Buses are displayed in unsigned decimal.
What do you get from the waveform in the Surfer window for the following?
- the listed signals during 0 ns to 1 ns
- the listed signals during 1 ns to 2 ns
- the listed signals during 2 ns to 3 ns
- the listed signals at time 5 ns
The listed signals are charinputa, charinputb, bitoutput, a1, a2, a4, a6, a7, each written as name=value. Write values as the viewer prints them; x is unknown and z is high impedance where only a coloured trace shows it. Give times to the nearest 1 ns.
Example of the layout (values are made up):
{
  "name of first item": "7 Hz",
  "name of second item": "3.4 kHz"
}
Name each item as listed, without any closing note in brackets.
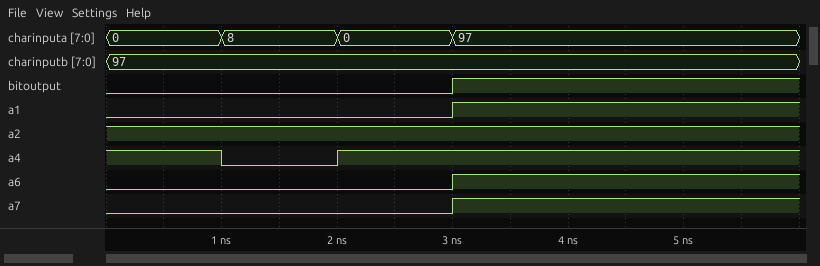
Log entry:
{
  "the listed signals during 0 ns to 1 ns": "charinputa=0, charinputb=97, bitoutput=0, a1=0, a2=1, a4=1, a6=0, a7=0",
  "the listed signals during 1 ns to 2 ns": "charinputa=8, charinputb=97, bitoutput=0, a1=0, a2=1, a4=0, a6=0, a7=0",
  "the listed signals during 2 ns to 3 ns": "charinputa=0, charinputb=97, bitoutput=0, a1=0, a2=1, a4=1, a6=0, a7=0",
  "the listed signals at time 5 ns": "charinputa=97, charinputb=97, bitoutput=1, a1=1, a2=1, a4=1, a6=1, a7=1"
}
